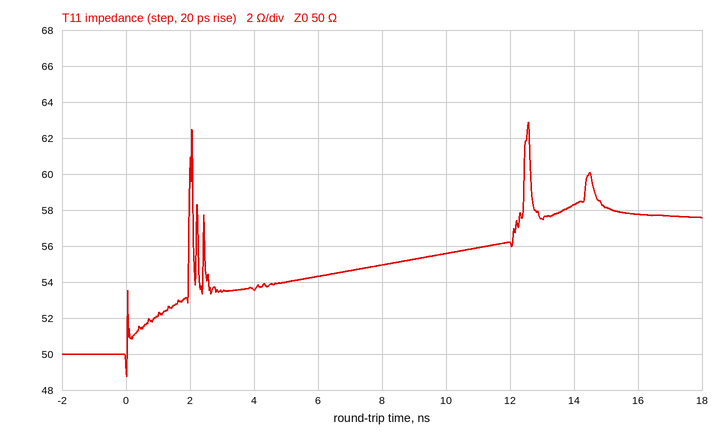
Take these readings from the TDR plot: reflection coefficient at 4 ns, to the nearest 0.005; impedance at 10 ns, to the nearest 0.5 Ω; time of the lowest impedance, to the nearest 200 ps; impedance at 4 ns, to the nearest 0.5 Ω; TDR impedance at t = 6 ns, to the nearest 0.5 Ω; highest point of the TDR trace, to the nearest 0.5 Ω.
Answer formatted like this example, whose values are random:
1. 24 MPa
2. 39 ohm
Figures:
1. +0.035
2. 55.5 Ω
3. 0.0 ns
4. 53.5 Ω
5. 54.5 Ω
6. 63.0 Ω
